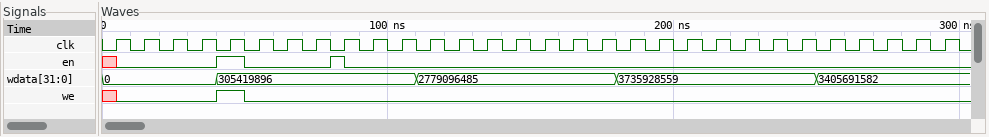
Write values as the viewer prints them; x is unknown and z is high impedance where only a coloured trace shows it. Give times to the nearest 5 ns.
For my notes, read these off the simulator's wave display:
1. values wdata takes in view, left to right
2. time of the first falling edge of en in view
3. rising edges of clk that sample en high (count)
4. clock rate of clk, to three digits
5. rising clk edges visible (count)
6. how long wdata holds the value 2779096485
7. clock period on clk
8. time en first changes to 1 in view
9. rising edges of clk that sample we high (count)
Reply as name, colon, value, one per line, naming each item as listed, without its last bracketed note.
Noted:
values wdata takes in view, left to right: 0, 305419896, 2779096485, 3735928559, 3405691582
time of the first falling edge of en in view: 50 ns
rising edges of clk that sample en high: 2
clock rate of clk, to three digits: 100 MHz
rising clk edges visible: 30
how long wdata holds the value 2779096485: 70 ns
clock period on clk: 10 ns
time en first changes to 1 in view: 40 ns
rising edges of clk that sample we high: 1
